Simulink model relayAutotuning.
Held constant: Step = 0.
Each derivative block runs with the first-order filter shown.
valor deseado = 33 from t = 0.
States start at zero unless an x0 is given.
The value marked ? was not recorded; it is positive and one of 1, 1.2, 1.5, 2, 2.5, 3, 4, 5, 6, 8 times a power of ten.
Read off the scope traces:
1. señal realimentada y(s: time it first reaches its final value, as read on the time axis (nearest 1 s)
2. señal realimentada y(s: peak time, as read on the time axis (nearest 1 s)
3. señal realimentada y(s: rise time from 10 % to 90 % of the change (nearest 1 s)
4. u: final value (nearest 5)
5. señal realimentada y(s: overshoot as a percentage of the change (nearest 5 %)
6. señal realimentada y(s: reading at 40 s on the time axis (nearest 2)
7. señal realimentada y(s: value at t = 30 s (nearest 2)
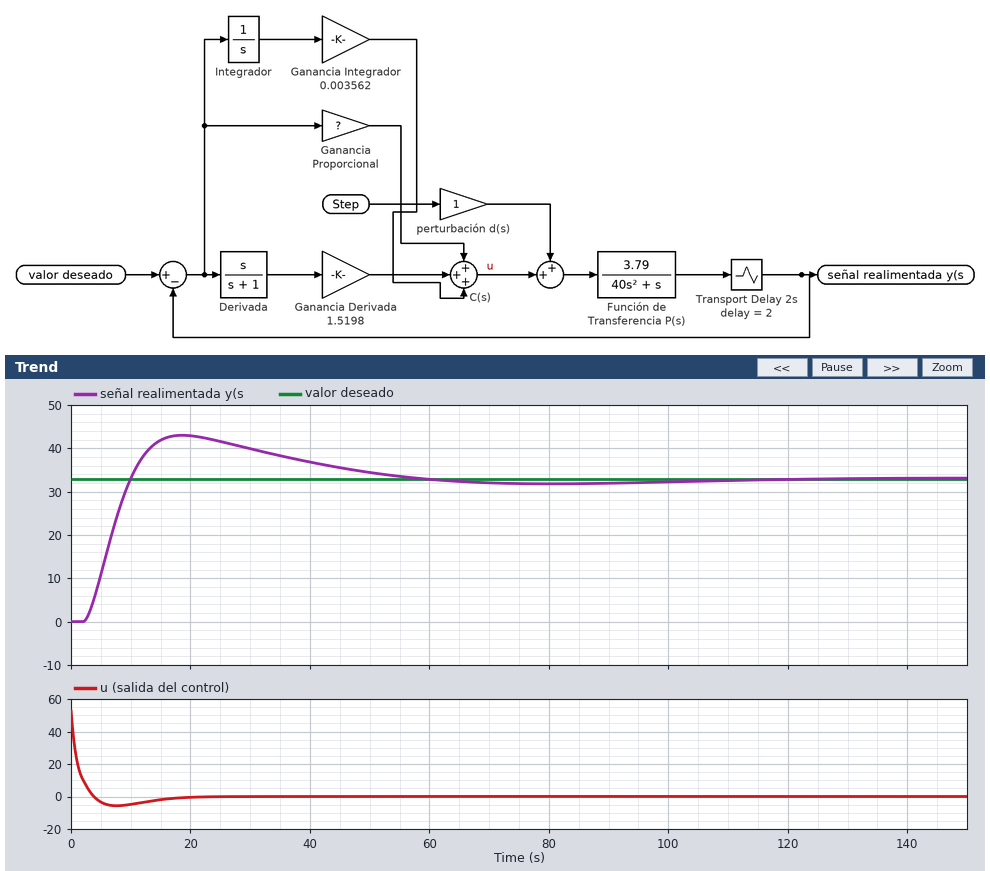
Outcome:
10 s
19 s
6 s
0
30 %
36
40
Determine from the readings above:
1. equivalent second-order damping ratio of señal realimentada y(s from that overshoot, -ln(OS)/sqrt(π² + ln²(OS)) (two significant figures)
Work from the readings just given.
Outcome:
0.36
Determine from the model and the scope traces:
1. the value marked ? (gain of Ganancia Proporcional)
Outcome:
0.1
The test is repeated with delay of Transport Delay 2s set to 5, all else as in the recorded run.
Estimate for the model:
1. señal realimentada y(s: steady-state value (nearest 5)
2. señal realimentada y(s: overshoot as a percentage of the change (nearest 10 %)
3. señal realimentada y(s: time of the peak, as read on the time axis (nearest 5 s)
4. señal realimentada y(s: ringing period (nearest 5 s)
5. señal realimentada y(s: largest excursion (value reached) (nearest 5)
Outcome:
35
90 %
20 s
35 s
60
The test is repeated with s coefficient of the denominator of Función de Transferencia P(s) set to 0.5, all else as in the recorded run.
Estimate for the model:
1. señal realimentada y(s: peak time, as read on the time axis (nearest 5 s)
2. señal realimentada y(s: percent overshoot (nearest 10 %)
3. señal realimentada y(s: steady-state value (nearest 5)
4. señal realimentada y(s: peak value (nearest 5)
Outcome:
20 s
40 %
35
45
